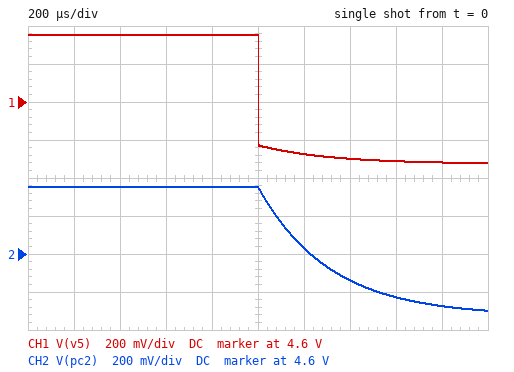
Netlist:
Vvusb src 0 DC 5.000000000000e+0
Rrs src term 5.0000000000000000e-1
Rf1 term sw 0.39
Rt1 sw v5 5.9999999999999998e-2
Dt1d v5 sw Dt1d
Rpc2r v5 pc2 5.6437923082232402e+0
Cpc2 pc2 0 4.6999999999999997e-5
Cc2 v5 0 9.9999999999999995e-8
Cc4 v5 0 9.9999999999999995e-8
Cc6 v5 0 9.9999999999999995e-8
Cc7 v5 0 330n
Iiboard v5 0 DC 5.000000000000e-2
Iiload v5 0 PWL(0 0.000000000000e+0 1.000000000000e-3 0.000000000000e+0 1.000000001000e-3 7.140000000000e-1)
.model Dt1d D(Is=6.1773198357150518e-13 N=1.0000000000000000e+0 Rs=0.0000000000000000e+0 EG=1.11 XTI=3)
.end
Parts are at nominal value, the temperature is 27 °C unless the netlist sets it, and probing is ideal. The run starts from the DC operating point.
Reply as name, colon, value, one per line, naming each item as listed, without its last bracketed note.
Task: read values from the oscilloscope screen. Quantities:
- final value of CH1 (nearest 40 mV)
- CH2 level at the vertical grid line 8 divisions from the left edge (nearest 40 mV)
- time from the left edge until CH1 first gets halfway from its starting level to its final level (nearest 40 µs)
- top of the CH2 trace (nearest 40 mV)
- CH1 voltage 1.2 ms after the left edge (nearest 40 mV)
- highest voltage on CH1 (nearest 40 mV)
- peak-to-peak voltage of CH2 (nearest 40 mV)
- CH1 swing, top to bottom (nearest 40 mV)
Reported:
final value of CH1: 4.28 V
CH2 level at the vertical grid line 8 divisions from the left edge: 4.36 V
time from the left edge until CH1 first gets halfway from its starting level to its final level: 1.00 ms
top of the CH2 trace: 4.96 V
CH1 voltage 1.2 ms after the left edge: 4.32 V
highest voltage on CH1: 4.96 V
peak-to-peak voltage of CH2: 640 mV
CH1 swing, top to bottom: 680 mV
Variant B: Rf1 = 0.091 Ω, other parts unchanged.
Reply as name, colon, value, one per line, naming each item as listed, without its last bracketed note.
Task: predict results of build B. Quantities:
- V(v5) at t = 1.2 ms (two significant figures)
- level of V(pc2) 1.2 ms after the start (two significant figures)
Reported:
V(v5) at t = 1.2 ms: 4.5 V
level of V(pc2) 1.2 ms after the start: 4.7 V
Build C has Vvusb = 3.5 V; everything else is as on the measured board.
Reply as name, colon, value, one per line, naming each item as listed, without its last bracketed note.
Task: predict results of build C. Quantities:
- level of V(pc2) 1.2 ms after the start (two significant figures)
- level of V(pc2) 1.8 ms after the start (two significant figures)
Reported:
level of V(pc2) 1.2 ms after the start: 3.1 V
level of V(pc2) 1.8 ms after the start: 2.8 V
